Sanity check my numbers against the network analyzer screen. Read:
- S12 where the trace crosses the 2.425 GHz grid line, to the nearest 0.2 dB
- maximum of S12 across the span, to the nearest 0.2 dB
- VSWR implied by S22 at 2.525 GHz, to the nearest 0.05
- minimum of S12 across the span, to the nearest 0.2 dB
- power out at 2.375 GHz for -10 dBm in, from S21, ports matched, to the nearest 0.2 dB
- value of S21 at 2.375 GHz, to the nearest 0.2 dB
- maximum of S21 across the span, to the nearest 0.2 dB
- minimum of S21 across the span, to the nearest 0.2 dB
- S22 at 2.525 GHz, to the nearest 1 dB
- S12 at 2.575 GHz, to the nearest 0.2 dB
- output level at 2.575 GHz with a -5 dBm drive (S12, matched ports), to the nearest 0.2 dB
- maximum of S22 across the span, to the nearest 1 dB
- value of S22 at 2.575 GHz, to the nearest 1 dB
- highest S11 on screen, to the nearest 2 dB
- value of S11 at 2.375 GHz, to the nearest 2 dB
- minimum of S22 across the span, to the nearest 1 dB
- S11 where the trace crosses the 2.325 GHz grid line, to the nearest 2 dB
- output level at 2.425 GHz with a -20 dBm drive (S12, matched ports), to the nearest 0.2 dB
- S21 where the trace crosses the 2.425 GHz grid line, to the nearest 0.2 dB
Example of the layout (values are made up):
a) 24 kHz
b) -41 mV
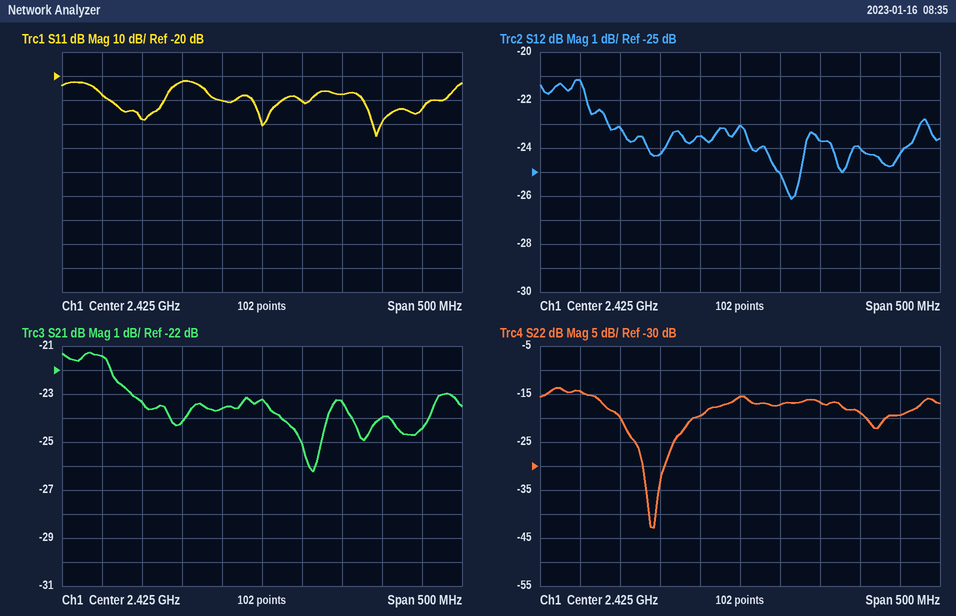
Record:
a) -23.0 dB
b) -21.2 dB
c) 1.35
d) -26.2 dB
e) -33.6 dBm
f) -23.6 dB
g) -21.2 dB
h) -26.2 dB
i) -17 dB
j) -24.0 dB
k) -29.0 dBm
l) -14 dB
m) -19 dB
n) -22 dB
o) -30 dB
p) -43 dB
q) -22 dB
r) -43.0 dBm
s) -23.2 dB
